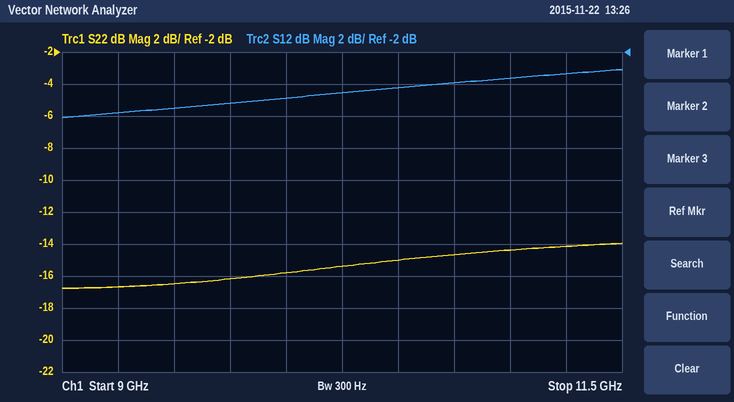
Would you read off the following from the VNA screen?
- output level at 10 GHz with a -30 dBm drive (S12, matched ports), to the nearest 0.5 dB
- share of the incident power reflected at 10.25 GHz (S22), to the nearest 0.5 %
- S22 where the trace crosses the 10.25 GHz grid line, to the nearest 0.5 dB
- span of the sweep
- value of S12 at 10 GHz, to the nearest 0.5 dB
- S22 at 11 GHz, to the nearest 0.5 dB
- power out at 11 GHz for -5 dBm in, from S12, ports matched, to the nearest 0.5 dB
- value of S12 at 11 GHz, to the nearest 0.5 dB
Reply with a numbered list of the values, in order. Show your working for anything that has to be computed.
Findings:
1. -30 dBm + (-5.0 dB) = -35.0 dBm
2. 10^(-15.5/10) ≈ 2.82 %, so 3.0 % to the nearest 0.5 %
3. -15.5 dB
4. 2.5 GHz
5. -5.0 dB
6. -14.5 dB
7. -5 dBm + (-3.5 dB) = -8.5 dBm
8. -3.5 dB
